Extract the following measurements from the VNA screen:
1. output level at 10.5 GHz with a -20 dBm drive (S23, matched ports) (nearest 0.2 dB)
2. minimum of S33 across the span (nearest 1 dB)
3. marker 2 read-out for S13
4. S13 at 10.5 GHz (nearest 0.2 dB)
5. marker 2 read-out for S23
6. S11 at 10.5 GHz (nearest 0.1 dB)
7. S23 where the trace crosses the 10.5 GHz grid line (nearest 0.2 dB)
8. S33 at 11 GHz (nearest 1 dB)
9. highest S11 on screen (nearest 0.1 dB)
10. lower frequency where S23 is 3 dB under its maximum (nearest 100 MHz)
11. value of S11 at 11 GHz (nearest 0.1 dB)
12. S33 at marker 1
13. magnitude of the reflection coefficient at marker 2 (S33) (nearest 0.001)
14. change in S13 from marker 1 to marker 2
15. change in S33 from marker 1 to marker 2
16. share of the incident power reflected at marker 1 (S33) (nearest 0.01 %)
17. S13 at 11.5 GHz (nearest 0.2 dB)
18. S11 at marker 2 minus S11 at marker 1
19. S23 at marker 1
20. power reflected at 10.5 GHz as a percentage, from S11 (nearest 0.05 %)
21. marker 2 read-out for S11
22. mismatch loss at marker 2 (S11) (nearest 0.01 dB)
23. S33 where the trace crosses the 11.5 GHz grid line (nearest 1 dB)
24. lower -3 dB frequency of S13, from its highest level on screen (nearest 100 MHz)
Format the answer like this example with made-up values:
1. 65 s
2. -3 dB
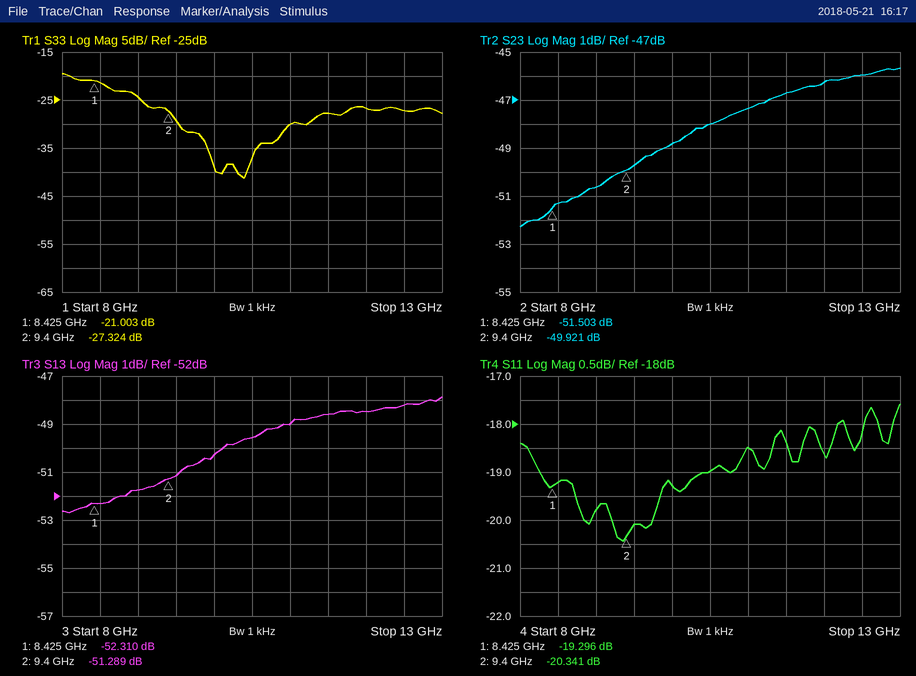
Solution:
1. -68.0 dBm
2. -41 dB
3. -51.289 dB
4. -49.6 dB
5. -49.921 dB
6. -19.0 dB
7. -48.0 dB
8. -30 dB
9. -17.6 dB
10. 10.1 GHz
11. -18.5 dB
12. -21.003 dB
13. 0.043
14. 1.021 dB
15. -6.321 dB
16. 0.79 %
17. -48.6 dB
18. -1.045 dB
19. -51.503 dB
20. 1.25 %
21. -20.341 dB
22. 0.04 dB
23. -28 dB
24. 9.6 GHz
